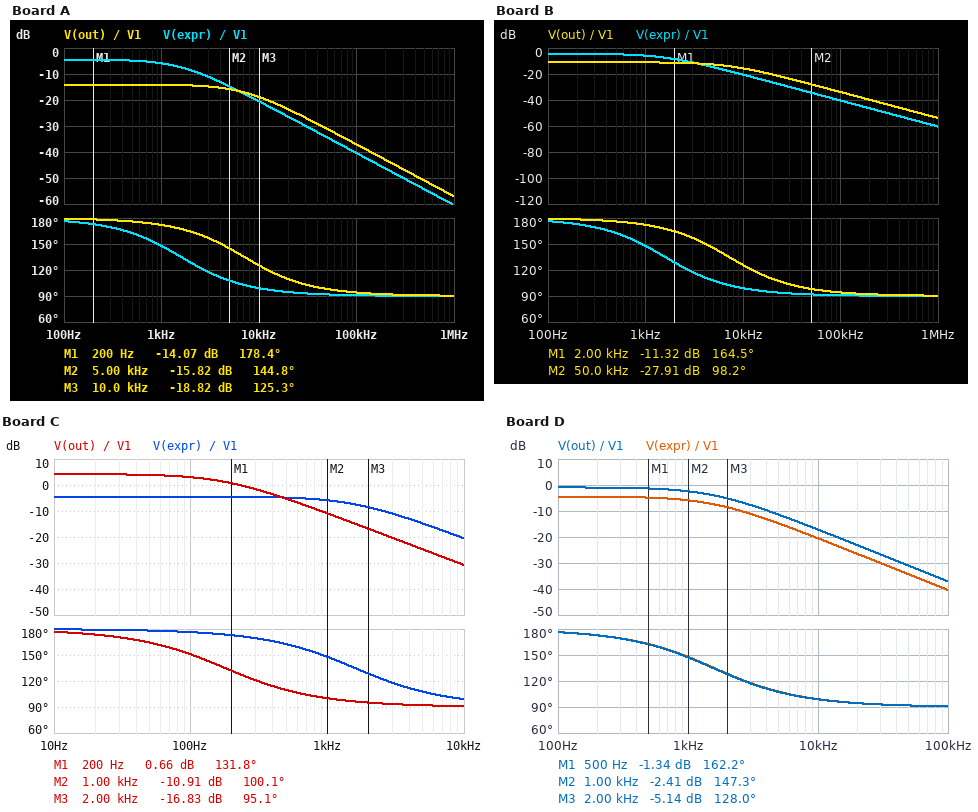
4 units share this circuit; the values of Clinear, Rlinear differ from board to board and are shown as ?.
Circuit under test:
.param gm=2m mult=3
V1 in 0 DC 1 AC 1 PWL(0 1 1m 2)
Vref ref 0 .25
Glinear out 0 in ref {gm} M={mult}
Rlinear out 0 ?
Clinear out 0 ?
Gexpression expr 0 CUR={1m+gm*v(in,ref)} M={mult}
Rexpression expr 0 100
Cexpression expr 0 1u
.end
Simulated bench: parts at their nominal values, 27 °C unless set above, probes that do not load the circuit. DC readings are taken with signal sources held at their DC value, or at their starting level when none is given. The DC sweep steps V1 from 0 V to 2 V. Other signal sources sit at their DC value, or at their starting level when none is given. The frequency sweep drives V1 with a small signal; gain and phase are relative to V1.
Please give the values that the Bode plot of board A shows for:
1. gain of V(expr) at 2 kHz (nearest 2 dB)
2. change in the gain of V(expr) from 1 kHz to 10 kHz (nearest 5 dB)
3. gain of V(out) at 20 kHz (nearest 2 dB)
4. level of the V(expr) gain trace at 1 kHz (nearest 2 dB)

-8 dB
-15 dB
-24 dB
-6 dB
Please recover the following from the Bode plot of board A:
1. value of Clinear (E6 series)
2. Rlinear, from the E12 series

680 nF
33 Ω
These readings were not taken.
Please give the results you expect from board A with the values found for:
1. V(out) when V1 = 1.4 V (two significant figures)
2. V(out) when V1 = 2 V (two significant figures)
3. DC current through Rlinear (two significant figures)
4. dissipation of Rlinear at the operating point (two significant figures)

-230 mV
-350 mV
4.5 mA
670 µW
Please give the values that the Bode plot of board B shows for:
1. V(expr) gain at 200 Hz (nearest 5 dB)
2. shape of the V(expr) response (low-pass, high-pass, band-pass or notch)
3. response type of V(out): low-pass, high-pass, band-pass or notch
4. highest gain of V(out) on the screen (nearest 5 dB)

-5 dB
low-pass
low-pass
-10 dB
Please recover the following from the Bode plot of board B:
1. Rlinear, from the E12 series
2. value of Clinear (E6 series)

47 Ω
470 nF
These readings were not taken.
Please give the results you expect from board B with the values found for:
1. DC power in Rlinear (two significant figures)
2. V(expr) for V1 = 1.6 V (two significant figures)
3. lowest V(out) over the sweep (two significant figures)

950 µW
-1.1 V
-490 mV
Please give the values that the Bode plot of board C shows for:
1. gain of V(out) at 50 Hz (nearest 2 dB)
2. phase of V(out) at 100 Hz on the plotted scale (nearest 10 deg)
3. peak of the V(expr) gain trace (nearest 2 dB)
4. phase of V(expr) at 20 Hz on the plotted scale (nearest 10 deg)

4 dB
150 deg
-4 dB
180 deg
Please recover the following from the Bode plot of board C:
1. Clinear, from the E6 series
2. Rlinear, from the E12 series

3.3 µF
270 Ω
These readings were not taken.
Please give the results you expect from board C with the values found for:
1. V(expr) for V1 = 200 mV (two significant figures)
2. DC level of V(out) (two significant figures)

-270 mV
-1.2 V
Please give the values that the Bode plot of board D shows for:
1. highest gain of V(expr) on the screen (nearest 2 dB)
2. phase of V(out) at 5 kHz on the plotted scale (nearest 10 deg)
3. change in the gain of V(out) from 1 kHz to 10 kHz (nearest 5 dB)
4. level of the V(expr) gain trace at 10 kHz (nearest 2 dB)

-4 dB
110 deg
-15 dB
-20 dB
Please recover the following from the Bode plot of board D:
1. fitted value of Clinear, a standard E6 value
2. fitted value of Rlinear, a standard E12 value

680 nF
150 Ω
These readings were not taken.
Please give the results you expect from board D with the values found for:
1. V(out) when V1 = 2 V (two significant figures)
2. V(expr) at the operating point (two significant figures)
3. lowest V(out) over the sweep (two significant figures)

-1.6 V
-750 mV
-1.6 V
